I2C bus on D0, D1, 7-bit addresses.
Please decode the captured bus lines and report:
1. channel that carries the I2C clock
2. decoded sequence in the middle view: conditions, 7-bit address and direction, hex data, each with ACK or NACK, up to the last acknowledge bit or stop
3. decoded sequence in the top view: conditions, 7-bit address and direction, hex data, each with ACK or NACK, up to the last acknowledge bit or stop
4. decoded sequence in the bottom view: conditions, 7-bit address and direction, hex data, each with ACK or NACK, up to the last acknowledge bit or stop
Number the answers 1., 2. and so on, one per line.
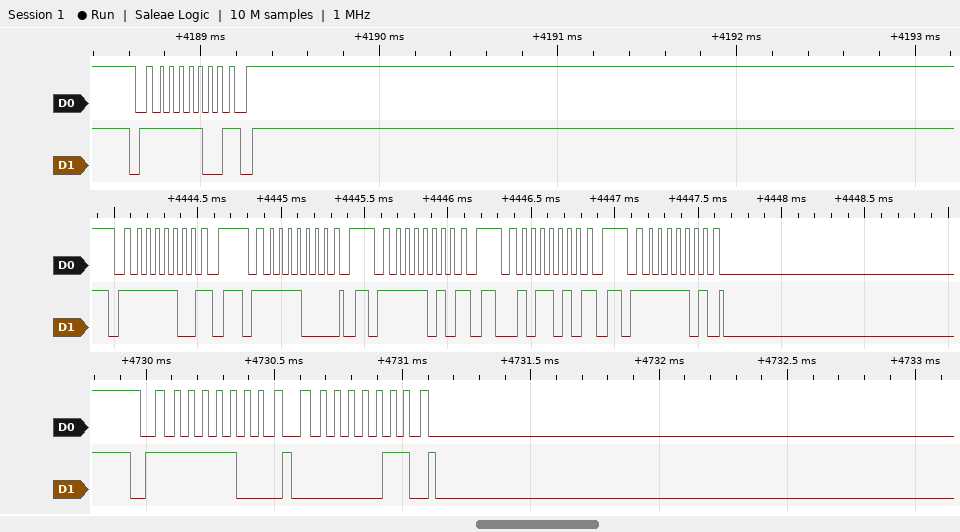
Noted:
1. D0
2. start, address 7E write NACK, stop, start, address 7C write ACK, stop, start, address 7D write NACK, stop, start, address 2D write NACK, stop, start, address 7E read ACK
3. start, address 7E write NACK, stop
4. start, address 7E write ACK, 03 ACK
